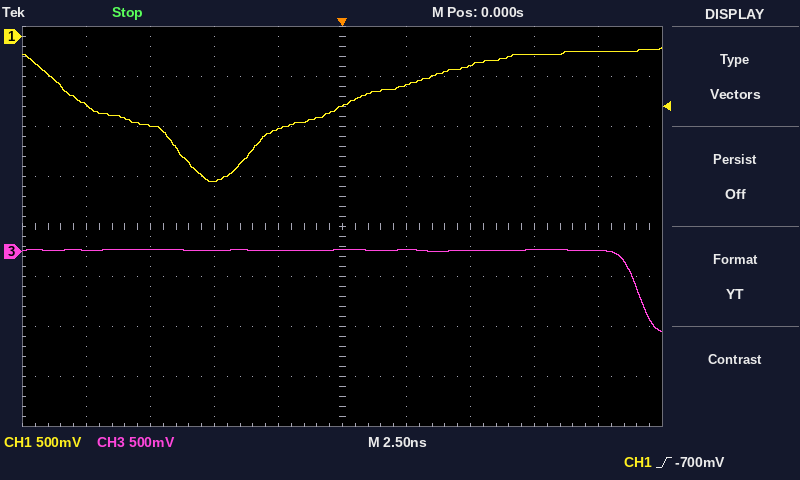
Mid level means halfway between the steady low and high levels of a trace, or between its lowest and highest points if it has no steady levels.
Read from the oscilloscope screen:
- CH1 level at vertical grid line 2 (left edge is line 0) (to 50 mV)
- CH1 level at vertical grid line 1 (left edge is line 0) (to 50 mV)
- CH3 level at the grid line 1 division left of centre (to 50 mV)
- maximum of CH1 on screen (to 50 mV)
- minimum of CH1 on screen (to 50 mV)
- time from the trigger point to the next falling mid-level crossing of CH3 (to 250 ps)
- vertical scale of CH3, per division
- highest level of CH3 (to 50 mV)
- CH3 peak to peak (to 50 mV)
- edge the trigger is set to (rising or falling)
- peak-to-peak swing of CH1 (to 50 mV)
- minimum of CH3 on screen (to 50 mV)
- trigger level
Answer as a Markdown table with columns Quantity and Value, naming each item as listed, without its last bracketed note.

| Quantity | Value |
|---|---|
| CH1 level at vertical grid line 2 (left edge is line 0) | -900 mV |
| CH1 level at vertical grid line 1 (left edge is line 0) | -700 mV |
| CH3 level at the grid line 1 division left of centre | 0 mV |
| maximum of CH1 on screen | -100 mV |
| minimum of CH1 on screen | -1.45 V |
| time from the trigger point to the next falling mid-level crossing of CH3 | 11.50 ns |
| vertical scale of CH3, per division | 500 mV |
| highest level of CH3 | 0 mV |
| CH3 peak to peak | 800 mV |
| edge the trigger is set to | rising |
| peak-to-peak swing of CH1 | 1.35 V |
| minimum of CH3 on screen | -800 mV |
| trigger level | -700 mV |
